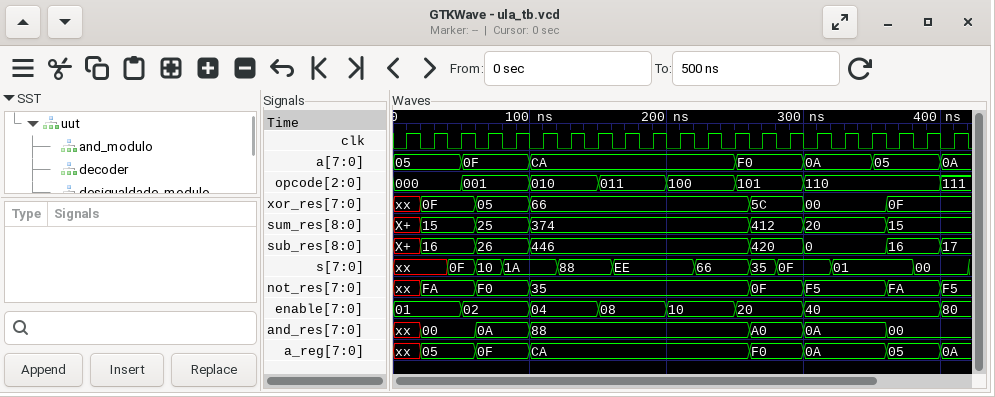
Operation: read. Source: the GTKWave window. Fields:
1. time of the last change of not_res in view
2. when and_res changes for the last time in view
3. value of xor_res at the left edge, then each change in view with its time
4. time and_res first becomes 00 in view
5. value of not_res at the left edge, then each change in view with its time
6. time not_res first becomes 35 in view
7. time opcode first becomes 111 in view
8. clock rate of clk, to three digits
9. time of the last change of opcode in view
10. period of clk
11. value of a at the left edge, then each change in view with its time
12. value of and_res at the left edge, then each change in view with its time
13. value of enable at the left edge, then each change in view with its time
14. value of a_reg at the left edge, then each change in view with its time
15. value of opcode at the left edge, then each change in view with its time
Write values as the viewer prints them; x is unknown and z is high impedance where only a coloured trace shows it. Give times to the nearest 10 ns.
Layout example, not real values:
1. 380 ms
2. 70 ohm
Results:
1. 400 ns
2. 360 ns
3. xx, 0F at 20 ns, 05 at 60 ns, 66 at 100 ns, 5C at 260 ns, 00 at 300 ns, 0F at 360 ns
4. 20 ns
5. xx, FA at 20 ns, F0 at 60 ns, 35 at 100 ns, 0F at 260 ns, F5 at 300 ns, FA at 360 ns, F5 at 400 ns
6. 100 ns
7. 400 ns
8. 50.0 MHz
9. 400 ns
10. 20 ns
11. 05, 0F at 50 ns, CA at 100 ns, F0 at 250 ns, 0A at 300 ns, 05 at 350 ns, 0A at 400 ns
12. xx, 00 at 20 ns, 0A at 60 ns, 88 at 100 ns, A0 at 260 ns, 0A at 300 ns, 00 at 360 ns
13. 01, 02 at 50 ns, 04 at 100 ns, 08 at 150 ns, 10 at 200 ns, 20 at 250 ns, 40 at 300 ns, 80 at 400 ns
14. xx, 05 at 20 ns, 0F at 60 ns, CA at 100 ns, F0 at 260 ns, 0A at 300 ns, 05 at 360 ns, 0A at 400 ns
15. 000, 001 at 50 ns, 010 at 100 ns, 011 at 150 ns, 100 at 200 ns, 101 at 250 ns, 110 at 300 ns, 111 at 400 ns
